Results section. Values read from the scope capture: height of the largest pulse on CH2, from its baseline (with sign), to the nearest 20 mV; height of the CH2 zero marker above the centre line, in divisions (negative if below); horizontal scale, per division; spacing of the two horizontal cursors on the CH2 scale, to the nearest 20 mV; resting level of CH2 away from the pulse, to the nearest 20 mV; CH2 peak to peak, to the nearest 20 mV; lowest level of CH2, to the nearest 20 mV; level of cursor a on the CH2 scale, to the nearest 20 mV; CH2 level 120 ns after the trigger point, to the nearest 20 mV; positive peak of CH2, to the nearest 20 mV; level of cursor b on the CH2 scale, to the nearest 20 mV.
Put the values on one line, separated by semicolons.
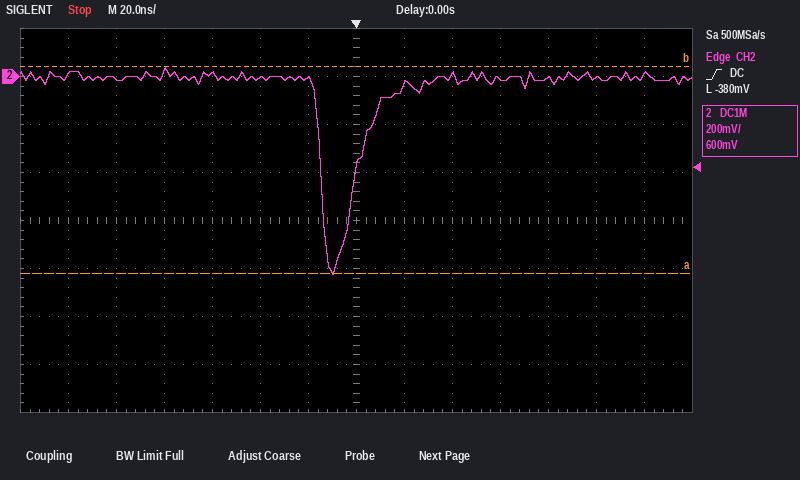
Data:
-820 mV; +3.0 div; 20 ns; 860 mV; 0 mV; 860 mV; -820 mV; -820 mV; 0 mV; 40 mV; 40 mV
